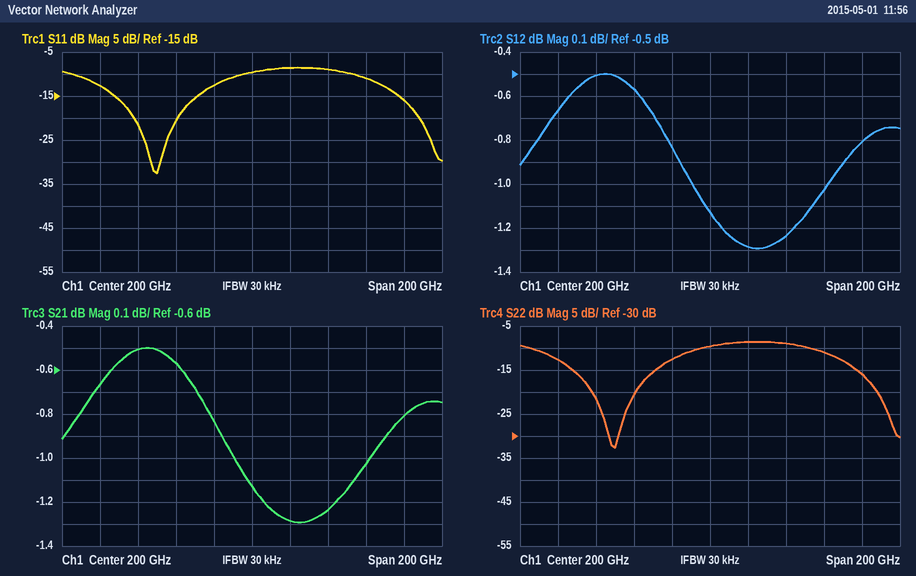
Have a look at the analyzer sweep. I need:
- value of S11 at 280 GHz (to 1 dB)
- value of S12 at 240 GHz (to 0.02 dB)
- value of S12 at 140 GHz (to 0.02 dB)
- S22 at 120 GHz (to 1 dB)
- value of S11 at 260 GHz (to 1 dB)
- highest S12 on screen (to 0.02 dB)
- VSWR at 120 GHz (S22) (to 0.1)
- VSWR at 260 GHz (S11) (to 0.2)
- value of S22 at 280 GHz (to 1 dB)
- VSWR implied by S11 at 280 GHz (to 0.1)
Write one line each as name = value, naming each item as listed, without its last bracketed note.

value of S11 at 280 GHz = -16 dB
value of S12 at 240 GHz = -1.24 dB
value of S12 at 140 GHz = -0.50 dB
S22 at 120 GHz = -13 dB
value of S11 at 260 GHz = -11 dB
highest S12 on screen = -0.50 dB
VSWR at 120 GHz (S22) = 1.6
VSWR at 260 GHz (S11) = 1.8
value of S22 at 280 GHz = -16 dB
VSWR implied by S11 at 280 GHz = 1.4
